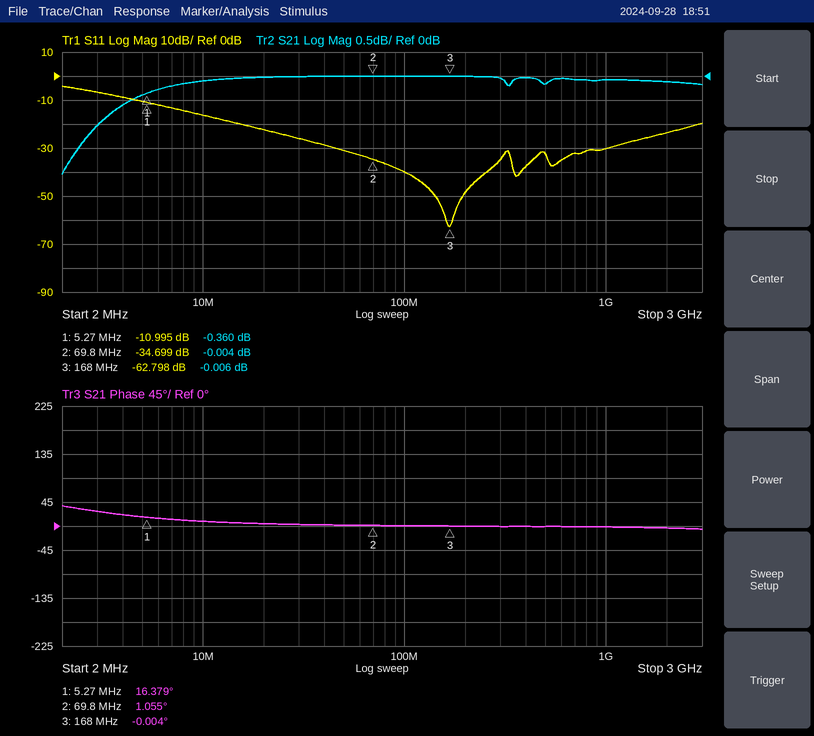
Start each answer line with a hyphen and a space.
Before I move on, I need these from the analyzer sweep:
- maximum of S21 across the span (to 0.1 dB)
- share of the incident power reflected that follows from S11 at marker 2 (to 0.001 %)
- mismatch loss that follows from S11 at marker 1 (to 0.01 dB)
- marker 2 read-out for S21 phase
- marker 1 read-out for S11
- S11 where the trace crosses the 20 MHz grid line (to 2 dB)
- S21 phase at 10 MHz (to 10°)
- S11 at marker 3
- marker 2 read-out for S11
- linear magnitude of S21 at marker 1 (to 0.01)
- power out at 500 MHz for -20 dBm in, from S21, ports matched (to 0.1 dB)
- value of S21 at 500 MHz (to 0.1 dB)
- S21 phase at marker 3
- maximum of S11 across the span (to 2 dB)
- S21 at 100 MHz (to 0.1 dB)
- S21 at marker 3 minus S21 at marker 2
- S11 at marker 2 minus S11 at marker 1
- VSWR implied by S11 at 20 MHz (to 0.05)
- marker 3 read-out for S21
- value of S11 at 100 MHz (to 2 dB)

- 0.0 dB
- 0.034 %
- 0.36 dB
- 1.055°
- -10.995 dB
- -22 dB
- 10°
- -62.798 dB
- -34.699 dB
- 0.96
- -20.2 dBm
- -0.2 dB
- -0.004°
- -4 dB
- 0.0 dB
- -0.002 dB
- -23.704 dB
- 1.15
- -0.006 dB
- -40 dB
